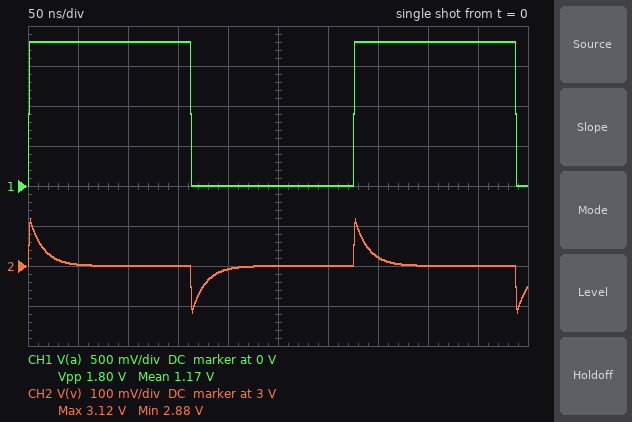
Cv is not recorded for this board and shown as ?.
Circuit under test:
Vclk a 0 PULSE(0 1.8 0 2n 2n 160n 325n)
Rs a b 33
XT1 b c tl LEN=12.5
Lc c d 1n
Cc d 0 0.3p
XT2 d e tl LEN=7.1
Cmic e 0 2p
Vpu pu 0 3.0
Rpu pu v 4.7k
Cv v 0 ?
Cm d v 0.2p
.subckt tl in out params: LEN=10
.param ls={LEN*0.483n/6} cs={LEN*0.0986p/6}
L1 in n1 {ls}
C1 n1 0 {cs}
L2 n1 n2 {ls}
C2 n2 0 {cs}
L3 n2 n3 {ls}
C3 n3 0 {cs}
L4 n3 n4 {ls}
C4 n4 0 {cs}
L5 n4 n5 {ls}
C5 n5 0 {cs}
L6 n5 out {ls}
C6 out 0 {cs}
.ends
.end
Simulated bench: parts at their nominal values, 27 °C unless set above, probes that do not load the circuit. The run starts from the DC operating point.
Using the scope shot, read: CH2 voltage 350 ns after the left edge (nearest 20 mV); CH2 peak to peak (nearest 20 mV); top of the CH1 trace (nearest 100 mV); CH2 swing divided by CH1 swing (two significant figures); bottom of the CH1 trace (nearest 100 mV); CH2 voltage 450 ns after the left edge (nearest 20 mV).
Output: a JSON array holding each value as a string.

["3.02 V", "240 mV", "1.8 V", "0.13", "0 V", "3.00 V"]
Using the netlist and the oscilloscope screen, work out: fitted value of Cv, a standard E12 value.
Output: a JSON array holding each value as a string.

["2.7 pF"]
